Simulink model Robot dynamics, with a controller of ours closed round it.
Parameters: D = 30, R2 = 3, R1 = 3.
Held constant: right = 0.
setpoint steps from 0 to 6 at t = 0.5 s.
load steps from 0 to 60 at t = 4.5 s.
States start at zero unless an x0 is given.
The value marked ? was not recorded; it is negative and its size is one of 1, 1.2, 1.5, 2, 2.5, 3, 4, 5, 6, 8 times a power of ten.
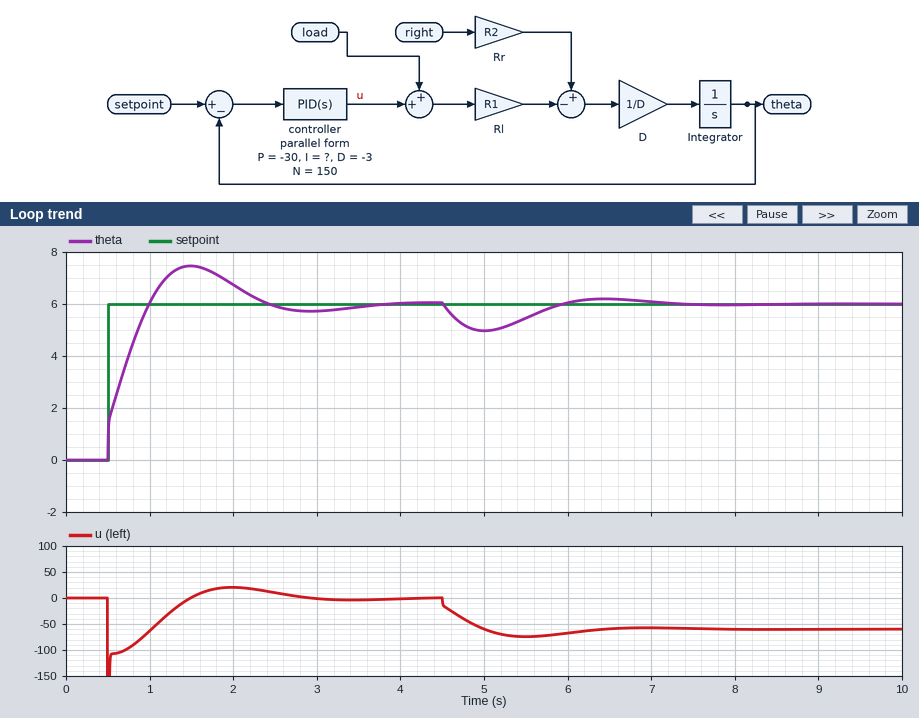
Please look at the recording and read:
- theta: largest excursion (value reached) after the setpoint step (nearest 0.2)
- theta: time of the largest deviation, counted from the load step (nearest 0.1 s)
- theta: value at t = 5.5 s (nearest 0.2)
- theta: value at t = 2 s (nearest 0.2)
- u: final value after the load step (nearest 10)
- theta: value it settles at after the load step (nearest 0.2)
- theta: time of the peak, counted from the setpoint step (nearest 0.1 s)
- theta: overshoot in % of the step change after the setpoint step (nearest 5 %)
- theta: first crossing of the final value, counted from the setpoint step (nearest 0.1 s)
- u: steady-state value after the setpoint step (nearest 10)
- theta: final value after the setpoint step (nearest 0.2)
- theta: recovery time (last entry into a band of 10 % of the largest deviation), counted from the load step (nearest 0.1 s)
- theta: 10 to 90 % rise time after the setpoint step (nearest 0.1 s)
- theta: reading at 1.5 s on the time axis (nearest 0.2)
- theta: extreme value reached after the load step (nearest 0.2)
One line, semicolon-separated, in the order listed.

7.4; 0.5 s; 5.4; 6.8; -60; 6.0; 1.0 s; 25 %; 0.5 s; 0; 6.0; 2.4 s; 0.4 s; 7.4; 5.0
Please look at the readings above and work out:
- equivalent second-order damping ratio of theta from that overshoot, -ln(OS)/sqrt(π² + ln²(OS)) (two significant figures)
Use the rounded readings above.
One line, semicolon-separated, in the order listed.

0.40
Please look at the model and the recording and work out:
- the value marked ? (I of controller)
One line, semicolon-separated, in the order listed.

-80
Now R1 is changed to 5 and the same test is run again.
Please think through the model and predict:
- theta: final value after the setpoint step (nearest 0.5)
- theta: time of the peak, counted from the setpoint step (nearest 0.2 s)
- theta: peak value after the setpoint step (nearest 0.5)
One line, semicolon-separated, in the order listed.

6.0; 0.8 s; 7.0
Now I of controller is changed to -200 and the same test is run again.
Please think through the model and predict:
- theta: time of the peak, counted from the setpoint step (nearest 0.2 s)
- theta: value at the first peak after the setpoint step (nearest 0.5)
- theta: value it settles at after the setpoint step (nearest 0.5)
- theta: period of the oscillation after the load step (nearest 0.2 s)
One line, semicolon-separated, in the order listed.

0.6 s; 8.0; 6.0; 1.6 s
